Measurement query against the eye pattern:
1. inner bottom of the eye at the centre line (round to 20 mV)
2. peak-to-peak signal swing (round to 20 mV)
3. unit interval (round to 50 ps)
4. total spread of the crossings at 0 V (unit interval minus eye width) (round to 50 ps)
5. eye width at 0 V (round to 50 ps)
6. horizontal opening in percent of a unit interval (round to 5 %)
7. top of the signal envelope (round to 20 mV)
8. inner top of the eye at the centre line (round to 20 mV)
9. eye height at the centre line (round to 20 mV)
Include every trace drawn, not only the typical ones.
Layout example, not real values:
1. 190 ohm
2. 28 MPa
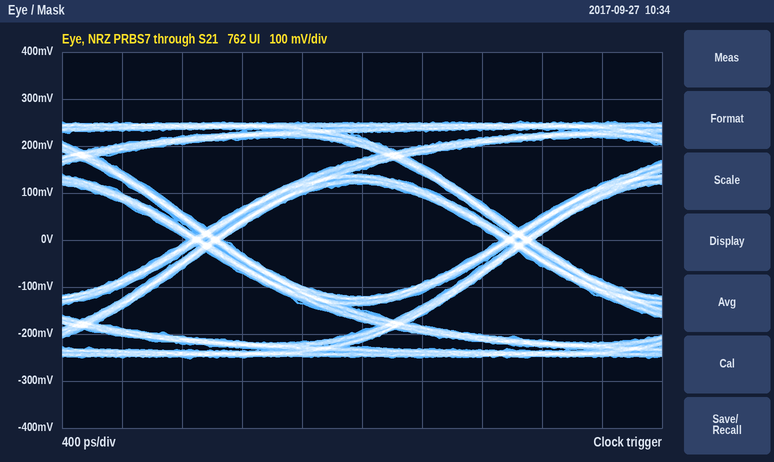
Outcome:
1. -120 mV
2. 500 mV
3. 2.10 ns
4. 250 ps
5. 1.85 ns
6. 90 %
7. 260 mV
8. 120 mV
9. 240 mV
